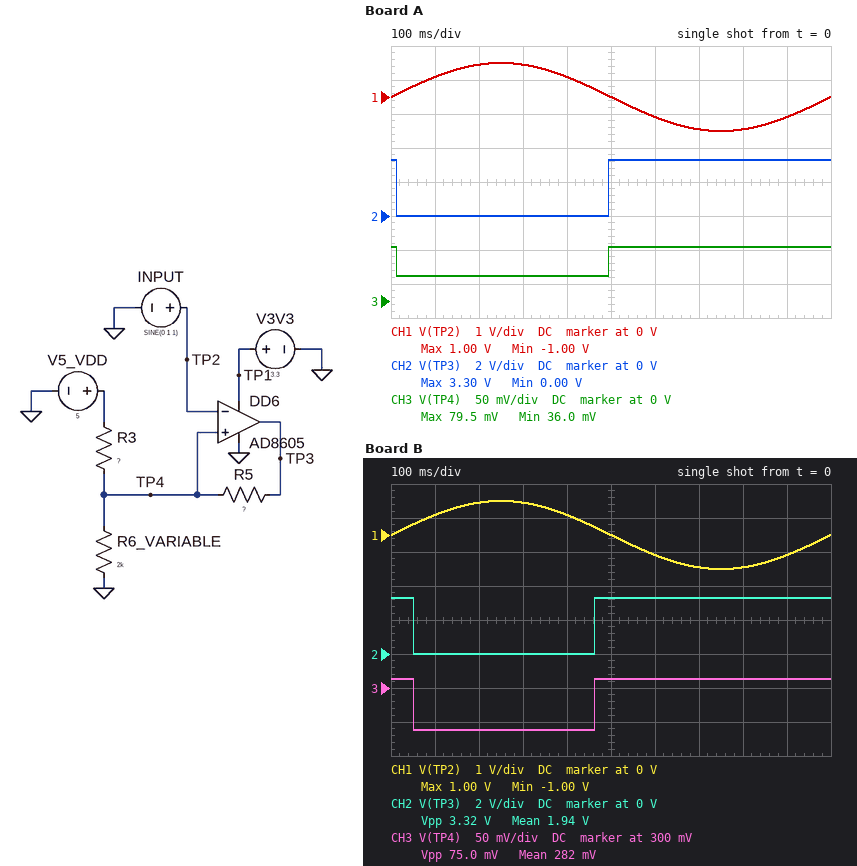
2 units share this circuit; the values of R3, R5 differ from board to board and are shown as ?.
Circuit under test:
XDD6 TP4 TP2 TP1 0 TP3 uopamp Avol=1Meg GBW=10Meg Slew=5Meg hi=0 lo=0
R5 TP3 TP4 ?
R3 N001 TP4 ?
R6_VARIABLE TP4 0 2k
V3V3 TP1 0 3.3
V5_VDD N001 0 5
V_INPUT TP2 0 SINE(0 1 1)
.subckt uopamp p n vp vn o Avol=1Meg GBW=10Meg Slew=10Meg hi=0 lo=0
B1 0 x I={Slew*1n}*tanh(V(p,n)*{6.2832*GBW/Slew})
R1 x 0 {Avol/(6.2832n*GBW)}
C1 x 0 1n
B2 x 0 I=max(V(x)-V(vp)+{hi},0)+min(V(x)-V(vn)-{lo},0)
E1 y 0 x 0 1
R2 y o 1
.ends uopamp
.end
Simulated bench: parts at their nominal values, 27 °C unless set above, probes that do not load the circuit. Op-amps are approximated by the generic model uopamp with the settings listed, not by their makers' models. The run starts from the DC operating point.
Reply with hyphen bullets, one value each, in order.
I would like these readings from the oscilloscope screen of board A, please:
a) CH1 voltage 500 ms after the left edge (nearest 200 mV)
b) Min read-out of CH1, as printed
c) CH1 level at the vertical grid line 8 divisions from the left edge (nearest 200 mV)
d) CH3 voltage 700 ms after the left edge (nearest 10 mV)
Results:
- 0 V
- -1.00 V
- -1.0 V
- 80 mV
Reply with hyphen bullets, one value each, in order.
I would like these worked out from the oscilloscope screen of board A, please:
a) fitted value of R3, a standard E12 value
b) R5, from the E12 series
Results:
- 270 kΩ
- 150 kΩ
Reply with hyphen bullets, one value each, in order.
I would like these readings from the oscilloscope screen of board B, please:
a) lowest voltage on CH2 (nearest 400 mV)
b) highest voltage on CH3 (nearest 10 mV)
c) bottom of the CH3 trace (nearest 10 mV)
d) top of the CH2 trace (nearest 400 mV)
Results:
- 0 V
- 310 mV
- 240 mV
- 3.2 V
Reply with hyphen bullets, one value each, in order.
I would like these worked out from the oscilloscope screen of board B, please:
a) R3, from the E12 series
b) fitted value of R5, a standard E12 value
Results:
- 39 kΩ
- 82 kΩ
